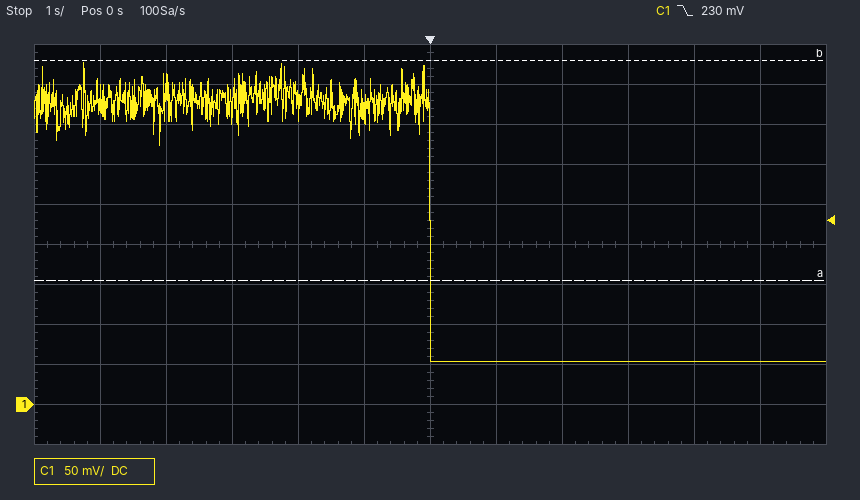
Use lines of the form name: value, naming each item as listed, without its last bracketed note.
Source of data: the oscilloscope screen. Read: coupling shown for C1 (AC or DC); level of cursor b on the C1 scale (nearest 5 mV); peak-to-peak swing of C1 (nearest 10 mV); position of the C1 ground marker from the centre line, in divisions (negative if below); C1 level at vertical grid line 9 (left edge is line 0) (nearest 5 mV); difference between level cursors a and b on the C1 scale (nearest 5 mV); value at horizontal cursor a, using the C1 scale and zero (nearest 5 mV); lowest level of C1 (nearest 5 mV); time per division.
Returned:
coupling shown for C1: DC
level of cursor b on the C1 scale: 430 mV
peak-to-peak swing of C1: 370 mV
position of the C1 ground marker from the centre line, in divisions: -4.0 div
C1 level at vertical grid line 9 (left edge is line 0): 55 mV
difference between level cursors a and b on the C1 scale: 275 mV
value at horizontal cursor a, using the C1 scale and zero: 155 mV
lowest level of C1: 55 mV
time per division: 1 s
